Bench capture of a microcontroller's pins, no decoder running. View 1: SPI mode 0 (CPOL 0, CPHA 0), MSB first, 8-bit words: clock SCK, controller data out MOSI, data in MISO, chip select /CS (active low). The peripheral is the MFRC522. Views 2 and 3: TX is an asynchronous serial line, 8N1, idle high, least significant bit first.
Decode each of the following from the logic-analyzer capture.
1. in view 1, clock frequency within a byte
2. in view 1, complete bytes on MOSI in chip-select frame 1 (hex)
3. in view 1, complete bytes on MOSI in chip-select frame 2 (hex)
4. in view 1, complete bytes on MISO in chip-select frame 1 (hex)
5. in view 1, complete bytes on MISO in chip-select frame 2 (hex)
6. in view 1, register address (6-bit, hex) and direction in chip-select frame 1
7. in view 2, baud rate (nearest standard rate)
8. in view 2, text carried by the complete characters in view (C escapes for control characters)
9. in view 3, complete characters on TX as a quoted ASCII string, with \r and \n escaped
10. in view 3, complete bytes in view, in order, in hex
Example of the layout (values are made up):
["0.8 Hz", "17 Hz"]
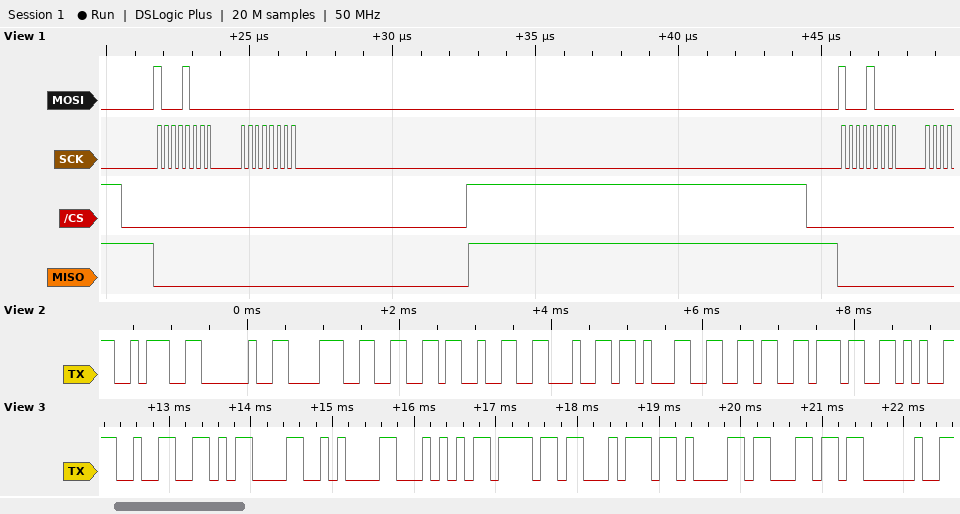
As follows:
["4 MHz", "0x88 0x00", "0x88", "0x00 0x00", "0x00", "0x04 read", "9600 baud", "\": 8f2d167\"", "\"2\\r\\nTotal \"", "32 0D 0A 54 6F 74 61 6C 20"]
